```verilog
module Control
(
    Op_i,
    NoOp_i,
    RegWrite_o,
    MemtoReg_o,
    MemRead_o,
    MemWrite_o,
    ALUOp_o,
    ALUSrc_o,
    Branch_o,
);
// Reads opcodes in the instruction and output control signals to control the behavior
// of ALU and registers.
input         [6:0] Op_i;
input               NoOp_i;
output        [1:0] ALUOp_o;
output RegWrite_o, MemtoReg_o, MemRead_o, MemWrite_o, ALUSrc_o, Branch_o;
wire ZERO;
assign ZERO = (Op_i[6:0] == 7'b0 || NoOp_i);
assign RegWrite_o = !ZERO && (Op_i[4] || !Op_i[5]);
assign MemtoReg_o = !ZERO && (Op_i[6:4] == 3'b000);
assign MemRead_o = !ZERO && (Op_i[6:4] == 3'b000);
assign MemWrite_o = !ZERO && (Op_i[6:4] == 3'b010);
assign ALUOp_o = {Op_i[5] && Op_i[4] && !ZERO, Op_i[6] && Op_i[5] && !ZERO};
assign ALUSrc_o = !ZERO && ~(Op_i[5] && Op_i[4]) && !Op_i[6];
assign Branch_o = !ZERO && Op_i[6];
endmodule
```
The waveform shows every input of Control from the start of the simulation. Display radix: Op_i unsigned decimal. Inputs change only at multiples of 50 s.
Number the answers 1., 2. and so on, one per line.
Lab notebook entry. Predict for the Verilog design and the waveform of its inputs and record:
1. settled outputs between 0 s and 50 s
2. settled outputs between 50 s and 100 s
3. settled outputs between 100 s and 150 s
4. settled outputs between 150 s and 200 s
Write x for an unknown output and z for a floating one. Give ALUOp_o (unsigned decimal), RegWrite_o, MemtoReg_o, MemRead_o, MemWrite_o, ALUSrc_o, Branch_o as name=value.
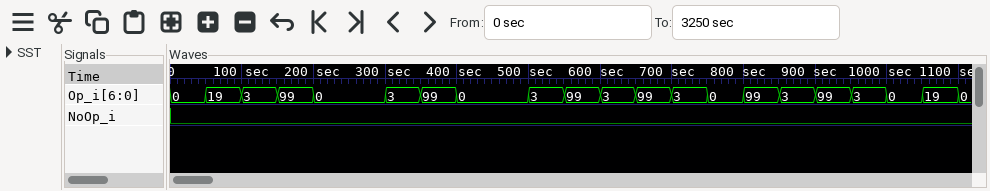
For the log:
1. ALUOp_o=0, RegWrite_o=0, MemtoReg_o=0, MemRead_o=0, MemWrite_o=0, ALUSrc_o=0, Branch_o=0
2. ALUOp_o=0, RegWrite_o=1, MemtoReg_o=0, MemRead_o=0, MemWrite_o=0, ALUSrc_o=1, Branch_o=0
3. ALUOp_o=0, RegWrite_o=1, MemtoReg_o=1, MemRead_o=1, MemWrite_o=0, ALUSrc_o=1, Branch_o=0
4. ALUOp_o=1, RegWrite_o=0, MemtoReg_o=0, MemRead_o=0, MemWrite_o=0, ALUSrc_o=0, Branch_o=1
